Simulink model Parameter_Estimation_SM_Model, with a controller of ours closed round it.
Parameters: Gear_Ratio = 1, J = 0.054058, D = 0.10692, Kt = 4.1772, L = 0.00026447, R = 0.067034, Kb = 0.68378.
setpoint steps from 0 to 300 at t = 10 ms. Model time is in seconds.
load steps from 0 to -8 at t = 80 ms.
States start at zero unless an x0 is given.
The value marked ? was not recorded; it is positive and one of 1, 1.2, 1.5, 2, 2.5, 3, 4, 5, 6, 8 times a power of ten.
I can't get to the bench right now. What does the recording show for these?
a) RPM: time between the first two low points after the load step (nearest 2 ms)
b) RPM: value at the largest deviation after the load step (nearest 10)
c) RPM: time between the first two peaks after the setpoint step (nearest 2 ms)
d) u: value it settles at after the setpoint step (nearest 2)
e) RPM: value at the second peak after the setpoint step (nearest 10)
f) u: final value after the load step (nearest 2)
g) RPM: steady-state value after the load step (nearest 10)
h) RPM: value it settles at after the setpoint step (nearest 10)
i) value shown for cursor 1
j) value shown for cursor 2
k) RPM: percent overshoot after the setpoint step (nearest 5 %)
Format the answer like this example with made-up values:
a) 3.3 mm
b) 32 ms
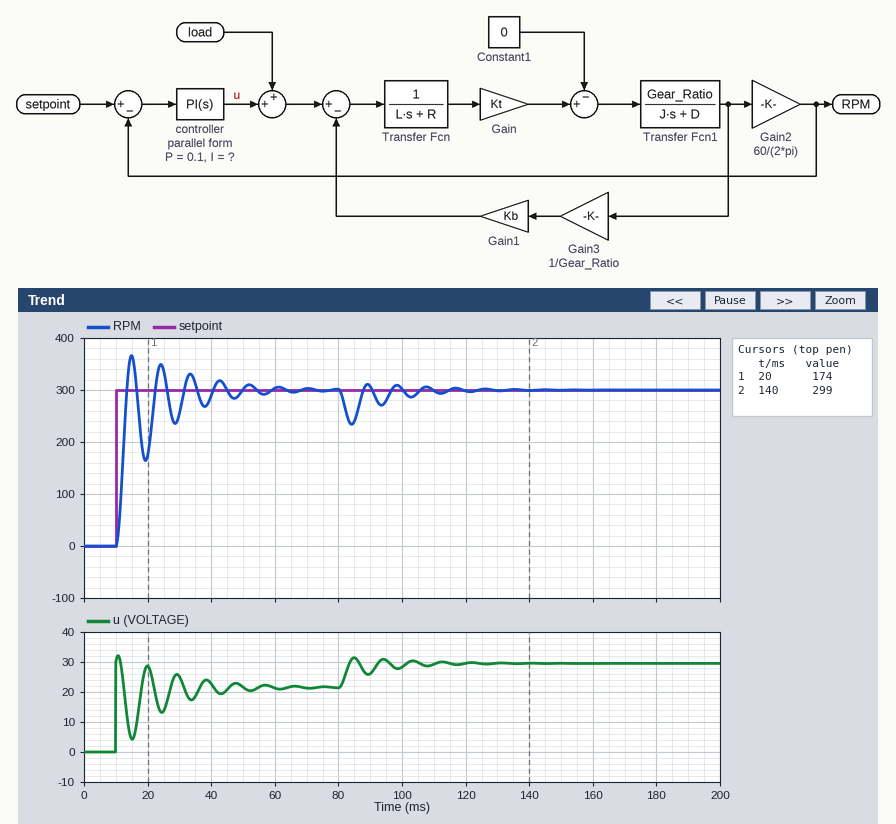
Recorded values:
a) 10 ms
b) 230
c) 10 ms
d) 22
e) 350
f) 30
g) 300
h) 300
i) 174
j) 299
k) 20 %
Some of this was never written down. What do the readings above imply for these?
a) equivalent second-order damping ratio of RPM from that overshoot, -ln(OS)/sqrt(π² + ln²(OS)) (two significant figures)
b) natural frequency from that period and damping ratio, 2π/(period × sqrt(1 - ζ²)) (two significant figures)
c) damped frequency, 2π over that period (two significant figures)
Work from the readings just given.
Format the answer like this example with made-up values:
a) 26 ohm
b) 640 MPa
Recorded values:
a) 0.46
b) 0.71 rad/ms
c) 0.63 rad/ms
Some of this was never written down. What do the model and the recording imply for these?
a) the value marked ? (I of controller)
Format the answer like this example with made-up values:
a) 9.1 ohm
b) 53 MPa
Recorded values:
a) 20
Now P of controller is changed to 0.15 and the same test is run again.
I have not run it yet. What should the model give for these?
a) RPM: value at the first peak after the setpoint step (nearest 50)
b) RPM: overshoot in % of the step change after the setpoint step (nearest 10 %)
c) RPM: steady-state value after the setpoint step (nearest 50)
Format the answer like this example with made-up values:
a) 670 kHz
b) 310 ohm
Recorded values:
a) 400
b) 30 %
c) 300
